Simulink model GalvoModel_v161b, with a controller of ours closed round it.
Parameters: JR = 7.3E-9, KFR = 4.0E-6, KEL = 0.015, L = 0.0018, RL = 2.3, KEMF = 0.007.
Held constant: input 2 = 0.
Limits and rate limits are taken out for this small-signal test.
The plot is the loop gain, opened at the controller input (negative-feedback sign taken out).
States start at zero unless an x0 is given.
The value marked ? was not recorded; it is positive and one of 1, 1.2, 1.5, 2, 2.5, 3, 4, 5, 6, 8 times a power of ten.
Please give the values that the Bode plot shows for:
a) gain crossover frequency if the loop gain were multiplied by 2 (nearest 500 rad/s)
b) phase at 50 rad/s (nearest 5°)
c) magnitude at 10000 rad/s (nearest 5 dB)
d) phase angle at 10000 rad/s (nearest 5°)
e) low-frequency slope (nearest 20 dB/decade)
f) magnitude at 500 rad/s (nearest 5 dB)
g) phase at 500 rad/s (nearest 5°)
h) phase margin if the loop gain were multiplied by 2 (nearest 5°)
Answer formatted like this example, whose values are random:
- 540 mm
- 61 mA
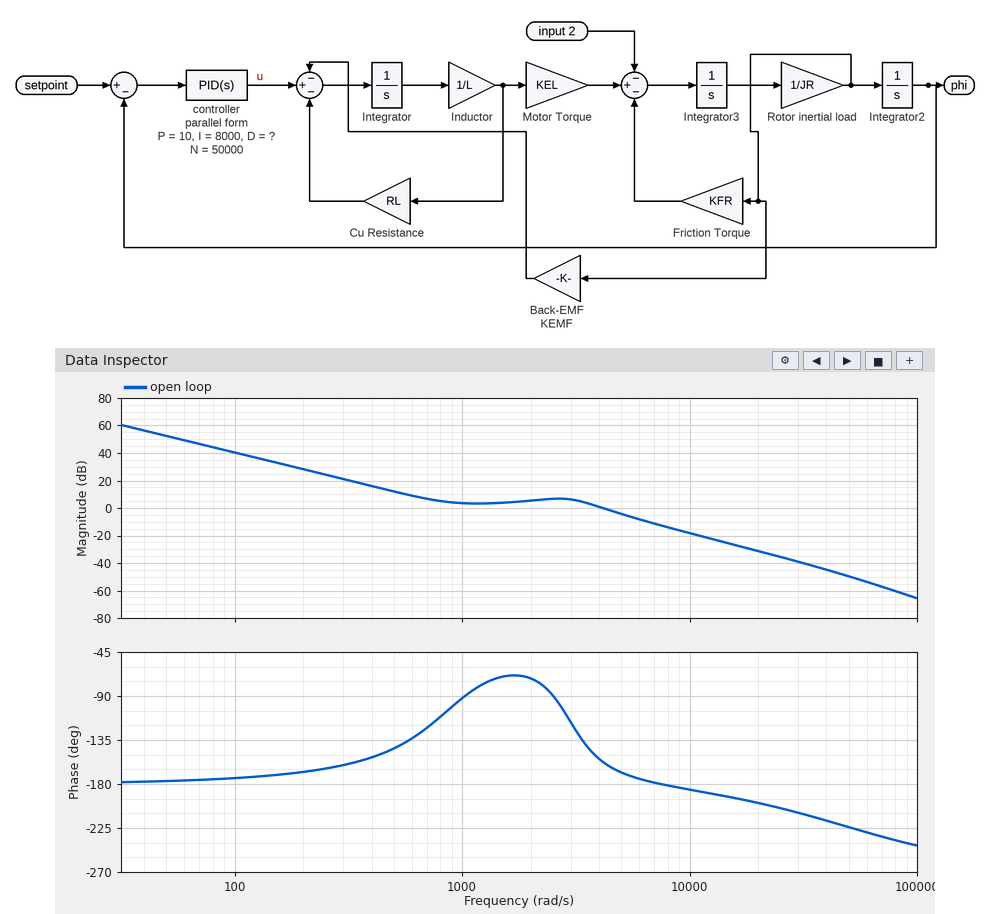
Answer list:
- 5500 rad/s
- -175°
- -20 dB
- -185°
- -40 dB/decade
- 10 dB
- -145°
- 10°
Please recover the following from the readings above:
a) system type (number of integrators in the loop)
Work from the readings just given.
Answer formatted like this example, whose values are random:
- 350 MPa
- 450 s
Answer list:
- 2
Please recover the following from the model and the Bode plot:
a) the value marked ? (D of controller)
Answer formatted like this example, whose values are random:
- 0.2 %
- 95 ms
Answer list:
- 0.01
